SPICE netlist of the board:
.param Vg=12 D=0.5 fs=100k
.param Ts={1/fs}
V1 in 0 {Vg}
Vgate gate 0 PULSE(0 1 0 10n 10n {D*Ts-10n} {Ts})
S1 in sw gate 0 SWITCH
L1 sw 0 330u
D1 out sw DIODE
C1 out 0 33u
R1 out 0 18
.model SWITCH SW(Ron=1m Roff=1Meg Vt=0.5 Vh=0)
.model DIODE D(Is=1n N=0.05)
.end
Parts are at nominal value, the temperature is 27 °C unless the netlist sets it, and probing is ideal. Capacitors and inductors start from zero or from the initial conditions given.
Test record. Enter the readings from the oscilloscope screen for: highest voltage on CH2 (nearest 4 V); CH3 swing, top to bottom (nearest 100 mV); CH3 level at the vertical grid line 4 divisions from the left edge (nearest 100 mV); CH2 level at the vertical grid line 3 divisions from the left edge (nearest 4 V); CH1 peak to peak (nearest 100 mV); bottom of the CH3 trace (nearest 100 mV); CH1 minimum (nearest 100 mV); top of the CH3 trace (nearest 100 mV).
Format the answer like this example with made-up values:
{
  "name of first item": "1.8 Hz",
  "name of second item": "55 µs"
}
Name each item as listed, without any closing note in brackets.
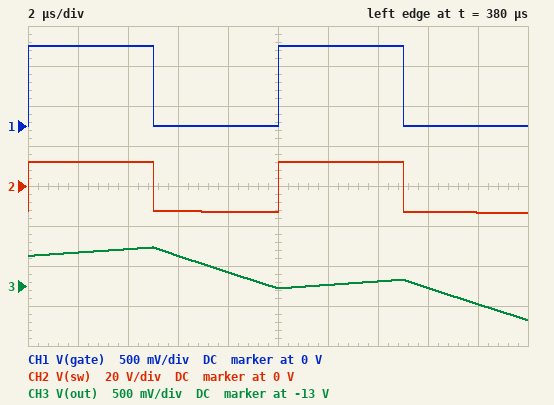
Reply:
{
  "highest voltage on CH2": "12 V",
  "CH3 swing, top to bottom": "900 mV",
  "CH3 level at the vertical grid line 4 divisions from the left edge": "-12.8 V",
  "CH2 level at the vertical grid line 3 divisions from the left edge": "-12 V",
  "CH1 peak to peak": "1.0 V",
  "bottom of the CH3 trace": "-13.4 V",
  "CH1 minimum": "0 V",
  "top of the CH3 trace": "-12.5 V"
}
